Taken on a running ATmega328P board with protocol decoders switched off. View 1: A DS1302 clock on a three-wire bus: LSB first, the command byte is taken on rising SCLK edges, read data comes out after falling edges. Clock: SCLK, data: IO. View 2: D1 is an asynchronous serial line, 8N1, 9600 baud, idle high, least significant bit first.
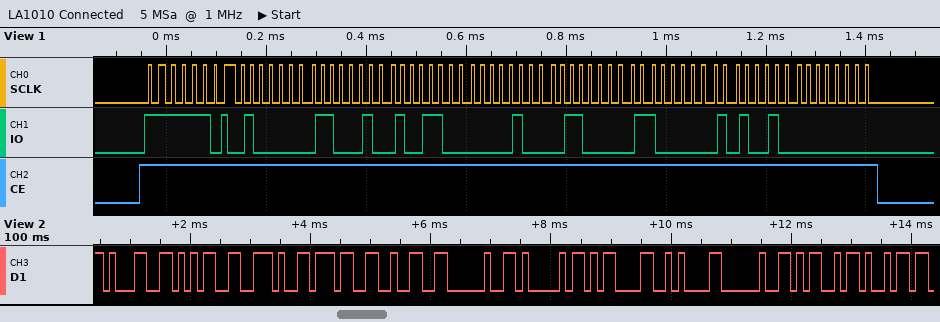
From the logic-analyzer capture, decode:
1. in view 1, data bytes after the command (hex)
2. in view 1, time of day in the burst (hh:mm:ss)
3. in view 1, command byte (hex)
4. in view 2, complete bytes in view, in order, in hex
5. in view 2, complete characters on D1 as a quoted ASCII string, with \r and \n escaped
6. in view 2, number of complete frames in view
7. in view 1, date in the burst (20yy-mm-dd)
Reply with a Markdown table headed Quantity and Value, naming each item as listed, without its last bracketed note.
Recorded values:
| Quantity | Value |
|---|---|
| in view 1, data bytes after the command | 02 23 19 10 06 03 25 00 |
| in view 1, time of day in the burst | 19:23:02 |
| in view 1, command byte | 0xBF |
| in view 2, complete bytes in view, in order, in hex | 31 35 2E 37 32 20 41 0D 0A 20 4D 69 |
| in view 2, complete characters on D1 as a quoted ASCII string, with \r and \n escaped | "15.72 A\r\n Mi" |
| in view 2, number of complete frames in view | 12 |
| in view 1, date in the burst | 2025-06-10 |
